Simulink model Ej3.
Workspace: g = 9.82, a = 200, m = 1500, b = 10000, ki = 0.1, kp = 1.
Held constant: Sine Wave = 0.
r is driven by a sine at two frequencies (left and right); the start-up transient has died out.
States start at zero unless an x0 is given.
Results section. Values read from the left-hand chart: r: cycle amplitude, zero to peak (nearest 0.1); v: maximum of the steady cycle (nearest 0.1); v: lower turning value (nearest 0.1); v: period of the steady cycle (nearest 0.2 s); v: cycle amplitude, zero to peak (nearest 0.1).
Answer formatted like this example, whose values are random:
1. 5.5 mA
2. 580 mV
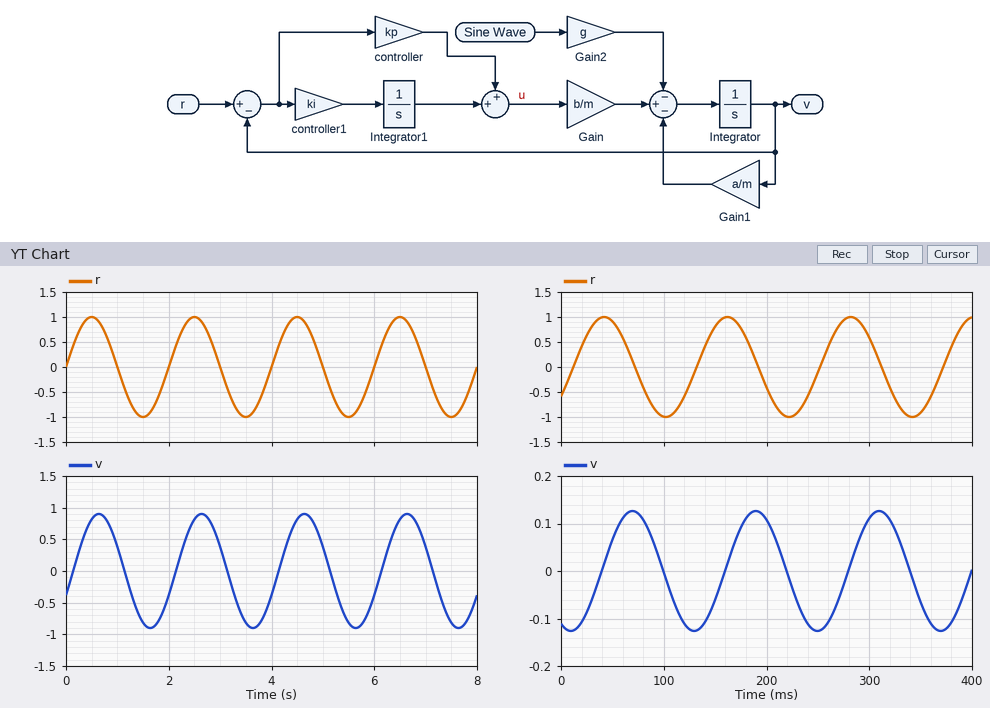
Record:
1. 1.0
2. 0.9
3. -0.9
4. 2.0 s
5. 0.9
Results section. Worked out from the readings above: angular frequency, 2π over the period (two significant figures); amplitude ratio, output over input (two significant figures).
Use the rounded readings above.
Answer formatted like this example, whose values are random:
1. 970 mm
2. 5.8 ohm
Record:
1. 3.1 rad/s
2. 0.90
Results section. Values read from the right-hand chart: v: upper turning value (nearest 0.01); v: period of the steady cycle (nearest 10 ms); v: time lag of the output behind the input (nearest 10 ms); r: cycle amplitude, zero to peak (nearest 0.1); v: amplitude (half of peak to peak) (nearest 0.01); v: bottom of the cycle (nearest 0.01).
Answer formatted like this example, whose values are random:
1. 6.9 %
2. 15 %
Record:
1. 0.13
2. 120 ms
3. 30 ms
4. 1.0
5. 0.13
6. -0.13
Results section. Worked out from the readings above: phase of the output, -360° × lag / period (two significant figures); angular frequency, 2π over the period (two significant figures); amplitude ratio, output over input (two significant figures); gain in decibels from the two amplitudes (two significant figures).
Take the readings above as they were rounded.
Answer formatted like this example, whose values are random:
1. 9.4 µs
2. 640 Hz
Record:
1. -90°
2. 0.052 rad/ms
3. 0.13
4. -18 dB
